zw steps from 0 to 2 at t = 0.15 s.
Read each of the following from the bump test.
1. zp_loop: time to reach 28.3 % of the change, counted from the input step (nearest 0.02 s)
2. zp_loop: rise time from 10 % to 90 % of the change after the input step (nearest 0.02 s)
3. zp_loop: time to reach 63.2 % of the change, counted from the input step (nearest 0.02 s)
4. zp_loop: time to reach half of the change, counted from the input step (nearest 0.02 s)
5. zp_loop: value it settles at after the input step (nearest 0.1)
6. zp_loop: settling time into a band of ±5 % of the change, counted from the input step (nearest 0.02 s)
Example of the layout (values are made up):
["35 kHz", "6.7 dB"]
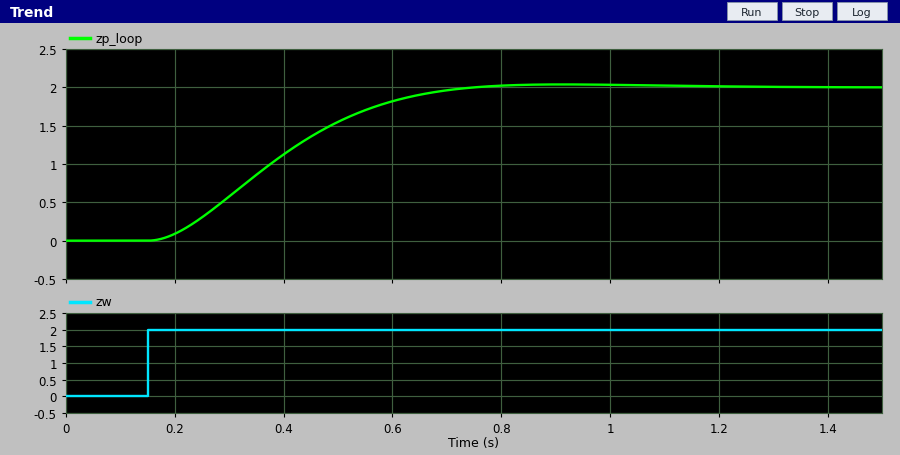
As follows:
["0.14 s", "0.36 s", "0.28 s", "0.22 s", "2.0", "0.50 s"]
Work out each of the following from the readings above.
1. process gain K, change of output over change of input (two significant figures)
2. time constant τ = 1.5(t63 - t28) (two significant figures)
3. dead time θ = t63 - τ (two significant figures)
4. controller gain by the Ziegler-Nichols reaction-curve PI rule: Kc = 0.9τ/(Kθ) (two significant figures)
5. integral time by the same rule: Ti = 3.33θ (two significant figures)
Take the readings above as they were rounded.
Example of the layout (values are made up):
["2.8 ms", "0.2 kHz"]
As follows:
["1.0", "0.21 s", "0.070 s", "2.7", "0.23 s"]
